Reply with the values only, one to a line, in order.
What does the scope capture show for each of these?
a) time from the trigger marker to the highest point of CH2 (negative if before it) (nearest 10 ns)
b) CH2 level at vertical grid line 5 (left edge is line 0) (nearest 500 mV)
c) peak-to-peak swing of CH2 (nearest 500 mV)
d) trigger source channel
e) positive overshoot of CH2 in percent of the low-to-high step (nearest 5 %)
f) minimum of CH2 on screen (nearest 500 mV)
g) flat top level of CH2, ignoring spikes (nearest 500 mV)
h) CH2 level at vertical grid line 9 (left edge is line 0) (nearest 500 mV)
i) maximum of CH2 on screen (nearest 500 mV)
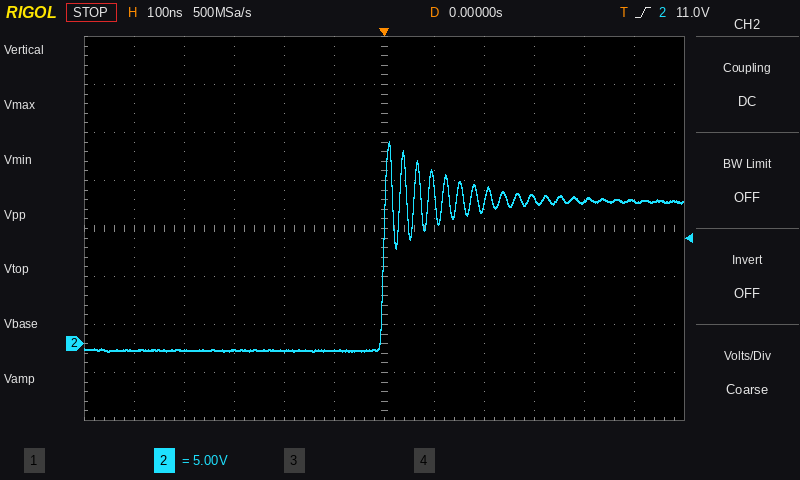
+10 ns
-500 mV
22.0 V
CH2
40 %
-1.0 V
15.0 V
15.0 V
21.0 V
